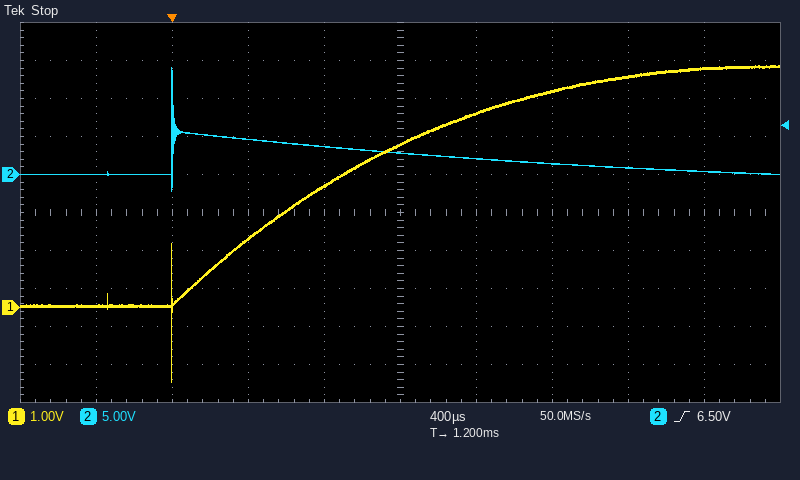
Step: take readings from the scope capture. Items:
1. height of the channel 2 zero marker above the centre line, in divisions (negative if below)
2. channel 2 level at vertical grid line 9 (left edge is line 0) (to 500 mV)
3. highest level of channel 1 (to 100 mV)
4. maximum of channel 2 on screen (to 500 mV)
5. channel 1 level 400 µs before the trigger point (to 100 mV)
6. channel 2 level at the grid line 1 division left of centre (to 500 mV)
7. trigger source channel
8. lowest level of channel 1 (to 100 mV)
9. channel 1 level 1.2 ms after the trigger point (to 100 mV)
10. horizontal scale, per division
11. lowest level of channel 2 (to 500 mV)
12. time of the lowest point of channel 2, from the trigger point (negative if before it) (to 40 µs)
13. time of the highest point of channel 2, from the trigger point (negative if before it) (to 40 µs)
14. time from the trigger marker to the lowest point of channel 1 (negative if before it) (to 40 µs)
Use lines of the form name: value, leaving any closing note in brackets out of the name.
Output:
height of the channel 2 zero marker above the centre line, in divisions: +1.0 div
channel 2 level at vertical grid line 9 (left edge is line 0): 500 mV
highest level of channel 1: 6.4 V
maximum of channel 2 on screen: 14.0 V
channel 1 level 400 µs before the trigger point: 0.0 V
channel 2 level at the grid line 1 division left of centre: 3.5 V
trigger source channel: channel 2
lowest level of channel 1: -2.0 V
channel 1 level 1.2 ms after the trigger point: 4.3 V
horizontal scale, per division: 400 µs
lowest level of channel 2: -2.0 V
time of the lowest point of channel 2, from the trigger point (negative if before it): 0 µs
time of the highest point of channel 2, from the trigger point (negative if before it): 0 µs
time from the trigger marker to the lowest point of channel 1 (negative if before it): 0 µs
